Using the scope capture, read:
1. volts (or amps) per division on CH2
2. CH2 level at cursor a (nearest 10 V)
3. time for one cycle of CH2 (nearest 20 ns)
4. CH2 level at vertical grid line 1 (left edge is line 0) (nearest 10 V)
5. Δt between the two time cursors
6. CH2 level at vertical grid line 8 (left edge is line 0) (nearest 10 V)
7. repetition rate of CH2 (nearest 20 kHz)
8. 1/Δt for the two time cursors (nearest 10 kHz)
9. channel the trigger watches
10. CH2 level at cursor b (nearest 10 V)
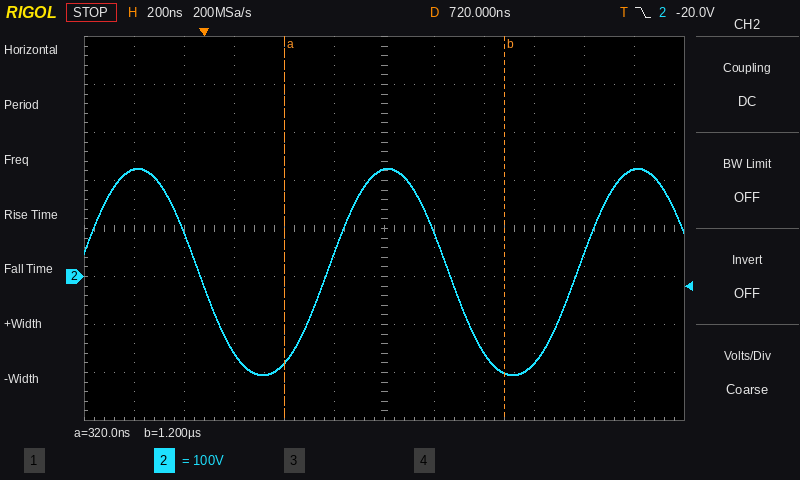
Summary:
100 V
-180 V
1.00 µs
220 V
880 ns
-160 V
1.00 MHz
1.14 MHz
CH2
-200 V
